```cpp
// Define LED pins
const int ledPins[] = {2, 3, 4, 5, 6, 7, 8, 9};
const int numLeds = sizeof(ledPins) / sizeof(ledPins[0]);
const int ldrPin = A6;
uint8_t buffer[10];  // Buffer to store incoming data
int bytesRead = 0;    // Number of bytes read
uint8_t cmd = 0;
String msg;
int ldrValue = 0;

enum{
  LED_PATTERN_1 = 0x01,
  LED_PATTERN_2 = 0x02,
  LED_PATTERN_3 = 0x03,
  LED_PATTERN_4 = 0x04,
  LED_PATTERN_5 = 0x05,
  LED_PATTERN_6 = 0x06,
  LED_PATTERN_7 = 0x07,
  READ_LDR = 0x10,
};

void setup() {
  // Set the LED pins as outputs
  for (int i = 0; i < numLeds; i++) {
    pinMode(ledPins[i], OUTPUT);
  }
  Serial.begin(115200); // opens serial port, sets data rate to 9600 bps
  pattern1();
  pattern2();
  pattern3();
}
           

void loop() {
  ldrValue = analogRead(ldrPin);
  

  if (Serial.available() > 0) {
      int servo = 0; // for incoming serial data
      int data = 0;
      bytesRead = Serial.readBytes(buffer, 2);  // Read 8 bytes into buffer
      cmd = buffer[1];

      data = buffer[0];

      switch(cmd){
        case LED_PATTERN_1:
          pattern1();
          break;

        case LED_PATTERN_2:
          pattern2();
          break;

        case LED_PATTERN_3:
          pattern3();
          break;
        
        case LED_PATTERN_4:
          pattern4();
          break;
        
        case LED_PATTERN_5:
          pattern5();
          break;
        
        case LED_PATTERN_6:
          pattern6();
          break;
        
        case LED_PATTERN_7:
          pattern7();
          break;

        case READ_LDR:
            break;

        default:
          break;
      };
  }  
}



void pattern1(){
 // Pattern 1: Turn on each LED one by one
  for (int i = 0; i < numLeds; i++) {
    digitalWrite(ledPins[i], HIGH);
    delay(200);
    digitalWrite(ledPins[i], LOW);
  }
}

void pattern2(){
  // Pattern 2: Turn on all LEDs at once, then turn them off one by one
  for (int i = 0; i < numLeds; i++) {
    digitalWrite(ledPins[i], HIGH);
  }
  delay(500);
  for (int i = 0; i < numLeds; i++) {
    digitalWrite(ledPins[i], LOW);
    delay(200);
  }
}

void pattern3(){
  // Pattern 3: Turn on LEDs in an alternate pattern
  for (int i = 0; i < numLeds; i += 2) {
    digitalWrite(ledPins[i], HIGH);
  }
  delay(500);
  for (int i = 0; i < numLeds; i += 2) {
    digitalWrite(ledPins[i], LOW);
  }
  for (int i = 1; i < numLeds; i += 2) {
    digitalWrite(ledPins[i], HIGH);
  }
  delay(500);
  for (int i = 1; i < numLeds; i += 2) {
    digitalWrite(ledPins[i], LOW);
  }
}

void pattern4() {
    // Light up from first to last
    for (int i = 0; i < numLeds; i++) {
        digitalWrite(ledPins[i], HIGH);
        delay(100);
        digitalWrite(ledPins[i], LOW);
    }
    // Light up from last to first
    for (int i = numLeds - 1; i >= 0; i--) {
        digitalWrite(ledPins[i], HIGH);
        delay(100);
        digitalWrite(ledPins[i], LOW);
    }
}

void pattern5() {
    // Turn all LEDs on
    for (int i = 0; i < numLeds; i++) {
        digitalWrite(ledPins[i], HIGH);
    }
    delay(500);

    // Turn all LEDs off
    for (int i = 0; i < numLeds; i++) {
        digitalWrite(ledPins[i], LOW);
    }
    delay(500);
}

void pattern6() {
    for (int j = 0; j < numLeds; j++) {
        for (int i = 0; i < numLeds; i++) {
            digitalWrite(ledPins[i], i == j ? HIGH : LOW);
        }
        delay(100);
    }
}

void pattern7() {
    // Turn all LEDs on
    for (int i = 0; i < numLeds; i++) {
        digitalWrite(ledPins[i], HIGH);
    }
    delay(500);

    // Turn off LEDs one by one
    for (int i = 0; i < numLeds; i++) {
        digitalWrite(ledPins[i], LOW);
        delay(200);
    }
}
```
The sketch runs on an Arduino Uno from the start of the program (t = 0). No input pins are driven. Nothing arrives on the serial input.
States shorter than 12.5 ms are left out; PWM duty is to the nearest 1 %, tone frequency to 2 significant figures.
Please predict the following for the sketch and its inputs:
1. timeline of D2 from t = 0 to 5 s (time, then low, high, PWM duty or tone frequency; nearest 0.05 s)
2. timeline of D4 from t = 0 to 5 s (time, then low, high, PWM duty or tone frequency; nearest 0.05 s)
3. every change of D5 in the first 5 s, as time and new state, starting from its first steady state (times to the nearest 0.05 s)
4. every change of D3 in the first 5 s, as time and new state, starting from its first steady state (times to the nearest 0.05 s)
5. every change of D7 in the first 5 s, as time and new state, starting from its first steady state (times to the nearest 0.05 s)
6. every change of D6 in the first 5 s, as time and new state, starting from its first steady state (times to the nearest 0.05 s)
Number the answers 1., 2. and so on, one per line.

1. 0 s high; 0.2 s low; 1.6 s high; 2.1 s low; 3.7 s high; 4.2 s low
2. 0 s low; 0.4 s high; 0.6 s low; 1.6 s high; 2.5 s low; 3.7 s high; 4.2 s low
3. 0 s low; 0.6 s high; 0.8 s low; 1.6 s high; 2.7 s low; 4.2 s high; 4.7 s low
4. 0 s low; 0.2 s high; 0.4 s low; 1.6 s high; 2.3 s low; 4.2 s high; 4.7 s low
5. 0 s low; 1 s high; 1.2 s low; 1.6 s high; 3.1 s low; 4.2 s high; 4.7 s low
6. 0 s low; 0.8 s high; 1 s low; 1.6 s high; 2.9 s low; 3.7 s high; 4.2 s low
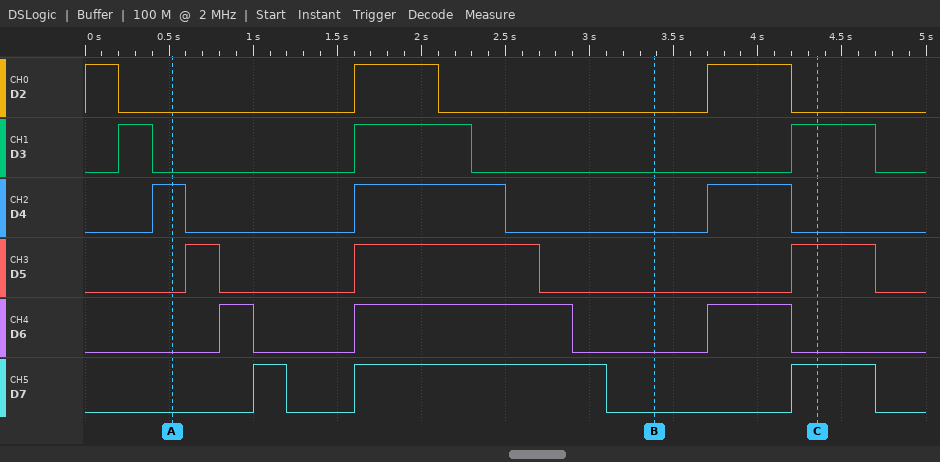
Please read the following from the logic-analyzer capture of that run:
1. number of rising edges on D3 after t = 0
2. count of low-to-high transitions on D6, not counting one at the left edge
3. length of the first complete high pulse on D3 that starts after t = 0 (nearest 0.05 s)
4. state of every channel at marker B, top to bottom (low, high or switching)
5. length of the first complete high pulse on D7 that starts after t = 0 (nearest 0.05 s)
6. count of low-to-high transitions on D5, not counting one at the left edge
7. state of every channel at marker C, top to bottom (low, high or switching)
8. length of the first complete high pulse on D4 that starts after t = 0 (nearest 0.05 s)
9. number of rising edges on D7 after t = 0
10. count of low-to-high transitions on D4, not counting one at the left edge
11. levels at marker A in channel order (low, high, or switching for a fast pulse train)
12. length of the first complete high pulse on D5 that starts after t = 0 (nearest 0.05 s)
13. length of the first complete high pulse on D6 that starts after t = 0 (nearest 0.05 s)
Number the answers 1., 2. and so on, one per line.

1. 3
2. 3
3. 0.20 s
4. D2 low, D3 low, D4 low, D5 low, D6 low, D7 low
5. 0.20 s
6. 3
7. D2 low, D3 high, D4 low, D5 high, D6 low, D7 high
8. 0.20 s
9. 3
10. 3
11. D2 low, D3 low, D4 high, D5 low, D6 low, D7 low
12. 0.20 s
13. 0.20 s
